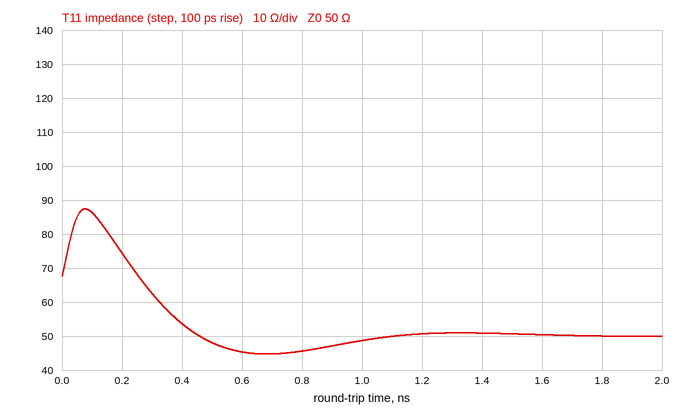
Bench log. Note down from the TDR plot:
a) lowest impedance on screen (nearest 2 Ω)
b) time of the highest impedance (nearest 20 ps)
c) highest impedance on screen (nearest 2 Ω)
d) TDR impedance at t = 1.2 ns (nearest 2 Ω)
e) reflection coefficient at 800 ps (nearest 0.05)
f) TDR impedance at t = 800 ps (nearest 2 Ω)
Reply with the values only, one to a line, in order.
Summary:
44 Ω
80 ps
88 Ω
50 Ω
-0.05
46 Ω
